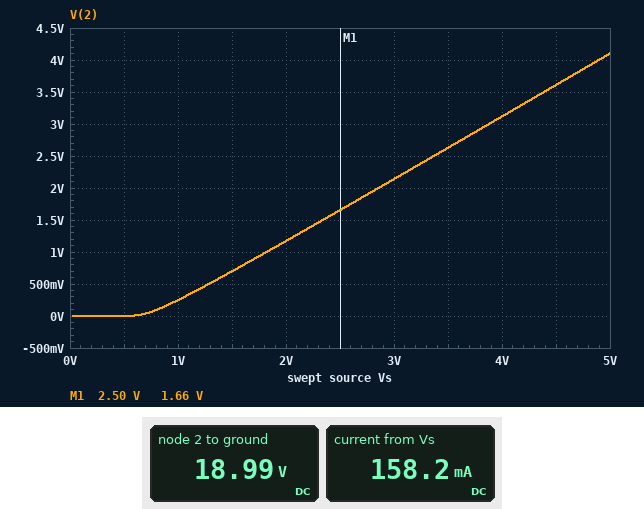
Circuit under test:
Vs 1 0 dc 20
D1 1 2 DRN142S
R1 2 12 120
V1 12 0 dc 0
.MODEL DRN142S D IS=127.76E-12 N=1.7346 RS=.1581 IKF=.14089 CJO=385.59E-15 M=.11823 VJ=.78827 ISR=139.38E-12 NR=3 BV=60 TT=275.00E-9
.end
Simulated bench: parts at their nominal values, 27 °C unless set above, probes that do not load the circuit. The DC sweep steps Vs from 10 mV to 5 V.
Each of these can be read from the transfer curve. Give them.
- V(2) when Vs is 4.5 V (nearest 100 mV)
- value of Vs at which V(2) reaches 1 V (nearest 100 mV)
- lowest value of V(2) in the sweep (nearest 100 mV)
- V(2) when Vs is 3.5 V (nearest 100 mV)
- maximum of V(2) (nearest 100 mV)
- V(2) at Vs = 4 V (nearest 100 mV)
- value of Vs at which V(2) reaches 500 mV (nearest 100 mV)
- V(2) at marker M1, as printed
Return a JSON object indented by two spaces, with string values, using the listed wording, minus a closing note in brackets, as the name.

{
  "V(2) when Vs is 4.5 V": "3.6 V",
  "value of Vs at which V(2) reaches 1 V": "1.8 V",
  "lowest value of V(2) in the sweep": "0 V",
  "V(2) when Vs is 3.5 V": "2.6 V",
  "maximum of V(2)": "4.1 V",
  "V(2) at Vs = 4 V": "3.1 V",
  "value of Vs at which V(2) reaches 500 mV": "1.3 V",
  "V(2) at marker M1, as printed": "1.66 V"
}
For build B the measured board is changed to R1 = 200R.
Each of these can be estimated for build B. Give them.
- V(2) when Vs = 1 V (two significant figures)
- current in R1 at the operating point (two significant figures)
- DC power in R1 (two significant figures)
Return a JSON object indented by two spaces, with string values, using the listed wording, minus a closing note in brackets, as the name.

{
  "V(2) when Vs = 1 V": "270 mV",
  "current in R1 at the operating point": "95 mA",
  "DC power in R1": "1.8 W"
}
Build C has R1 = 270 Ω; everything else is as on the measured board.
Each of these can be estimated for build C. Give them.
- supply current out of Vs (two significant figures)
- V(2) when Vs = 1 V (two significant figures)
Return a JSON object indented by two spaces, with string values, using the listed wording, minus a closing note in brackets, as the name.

{
  "supply current out of Vs": "71 mA",
  "V(2) when Vs = 1 V": "280 mV"
}
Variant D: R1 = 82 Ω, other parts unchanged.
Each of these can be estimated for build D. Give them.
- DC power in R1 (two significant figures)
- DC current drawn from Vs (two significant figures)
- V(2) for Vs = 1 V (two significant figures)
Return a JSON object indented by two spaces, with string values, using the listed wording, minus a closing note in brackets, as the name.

{
  "DC power in R1": "4.4 W",
  "DC current drawn from Vs": "230 mA",
  "V(2) for Vs = 1 V": "230 mV"
}
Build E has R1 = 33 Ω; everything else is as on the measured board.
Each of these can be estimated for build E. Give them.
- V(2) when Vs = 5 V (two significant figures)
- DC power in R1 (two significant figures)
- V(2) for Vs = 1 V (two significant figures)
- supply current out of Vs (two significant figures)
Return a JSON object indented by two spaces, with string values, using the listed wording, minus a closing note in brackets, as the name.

{
  "V(2) when Vs = 5 V": "4.0 V",
  "DC power in R1": "11 W",
  "V(2) for Vs = 1 V": "200 mV",
  "supply current out of Vs": "570 mA"
}
